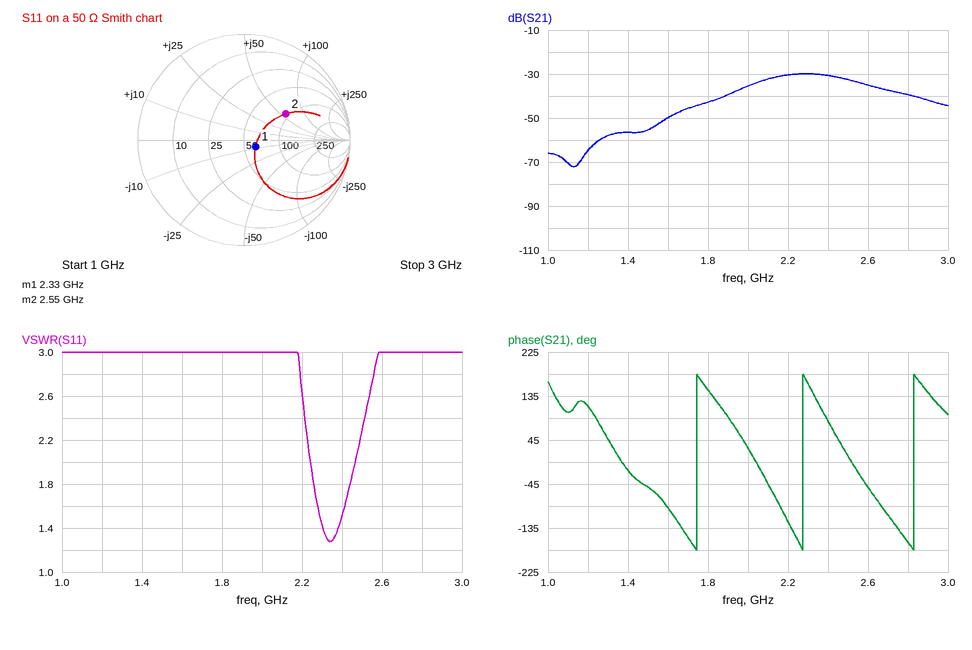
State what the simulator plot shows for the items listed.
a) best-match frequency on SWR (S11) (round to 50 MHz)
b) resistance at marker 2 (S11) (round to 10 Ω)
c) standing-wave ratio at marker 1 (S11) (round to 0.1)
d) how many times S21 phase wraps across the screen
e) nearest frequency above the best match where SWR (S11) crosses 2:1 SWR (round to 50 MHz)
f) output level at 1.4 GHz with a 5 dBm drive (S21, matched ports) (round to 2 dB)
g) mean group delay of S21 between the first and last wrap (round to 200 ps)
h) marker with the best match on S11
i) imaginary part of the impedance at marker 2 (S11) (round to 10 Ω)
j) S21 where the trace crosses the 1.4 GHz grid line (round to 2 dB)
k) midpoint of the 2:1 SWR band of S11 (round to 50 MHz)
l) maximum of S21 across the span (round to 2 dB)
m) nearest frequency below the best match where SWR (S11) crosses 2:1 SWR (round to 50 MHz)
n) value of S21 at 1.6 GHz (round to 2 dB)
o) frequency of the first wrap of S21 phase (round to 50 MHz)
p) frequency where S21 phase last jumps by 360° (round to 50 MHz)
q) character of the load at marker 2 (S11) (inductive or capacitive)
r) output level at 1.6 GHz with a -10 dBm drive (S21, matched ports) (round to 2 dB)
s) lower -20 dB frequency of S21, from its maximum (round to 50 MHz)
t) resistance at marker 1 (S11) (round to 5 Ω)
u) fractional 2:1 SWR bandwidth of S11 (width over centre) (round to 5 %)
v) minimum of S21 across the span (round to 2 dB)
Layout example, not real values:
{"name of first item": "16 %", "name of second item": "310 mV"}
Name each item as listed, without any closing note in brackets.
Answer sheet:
{"best-match frequency on SWR (S11)": "2.35 GHz", "resistance at marker 2 (S11)": "90 Ω", "standing-wave ratio at marker 1 (S11)": "1.3", "how many times S21 phase wraps across the screen": "3", "nearest frequency above the best match where SWR (S11) crosses 2:1 SWR": "2.45 GHz", "output level at 1.4 GHz with a 5 dBm drive (S21, matched ports)": "-52 dBm", "mean group delay of S21 between the first and last wrap": "1.8 ns", "marker with the best match on S11": "marker 1", "imaginary part of the impedance at marker 2 (S11)": "+60 Ω", "S21 where the trace crosses the 1.4 GHz grid line": "-56 dB", "midpoint of the 2:1 SWR band of S11": "2.35 GHz", "maximum of S21 across the span": "-30 dB", "nearest frequency below the best match where SWR (S11) crosses 2:1 SWR": "2.25 GHz", "value of S21 at 1.6 GHz": "-50 dB", "frequency of the first wrap of S21 phase": "1.75 GHz", "frequency where S21 phase last jumps by 360°": "2.85 GHz", "character of the load at marker 2 (S11)": "inductive", "output level at 1.6 GHz with a -10 dBm drive (S21, matched ports)": "-60 dBm", "lower -20 dB frequency of S21, from its maximum": "1.60 GHz", "resistance at marker 1 (S11)": "60 Ω", "fractional 2:1 SWR bandwidth of S11 (width over centre)": "10 %", "minimum of S21 across the span": "-72 dB"}
